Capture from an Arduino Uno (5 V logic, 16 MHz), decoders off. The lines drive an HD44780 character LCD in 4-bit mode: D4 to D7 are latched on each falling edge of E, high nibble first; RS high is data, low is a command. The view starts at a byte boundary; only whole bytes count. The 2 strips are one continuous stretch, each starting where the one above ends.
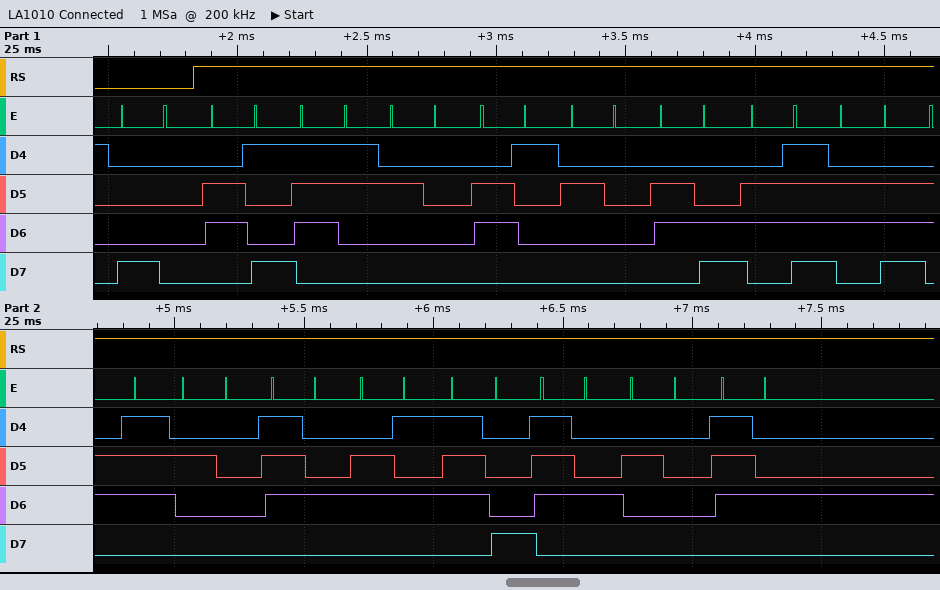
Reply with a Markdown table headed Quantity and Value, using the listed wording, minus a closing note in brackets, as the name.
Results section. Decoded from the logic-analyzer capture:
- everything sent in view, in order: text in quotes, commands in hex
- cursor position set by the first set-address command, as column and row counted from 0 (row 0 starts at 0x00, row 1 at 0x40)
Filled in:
| Quantity | Value |
|---|---|
| everything sent in view, in order: text in quotes, commands in hex | 0x80 "is a long text t" |
| cursor position set by the first set-address command, as column and row counted from 0 | column 0, row 0 |
